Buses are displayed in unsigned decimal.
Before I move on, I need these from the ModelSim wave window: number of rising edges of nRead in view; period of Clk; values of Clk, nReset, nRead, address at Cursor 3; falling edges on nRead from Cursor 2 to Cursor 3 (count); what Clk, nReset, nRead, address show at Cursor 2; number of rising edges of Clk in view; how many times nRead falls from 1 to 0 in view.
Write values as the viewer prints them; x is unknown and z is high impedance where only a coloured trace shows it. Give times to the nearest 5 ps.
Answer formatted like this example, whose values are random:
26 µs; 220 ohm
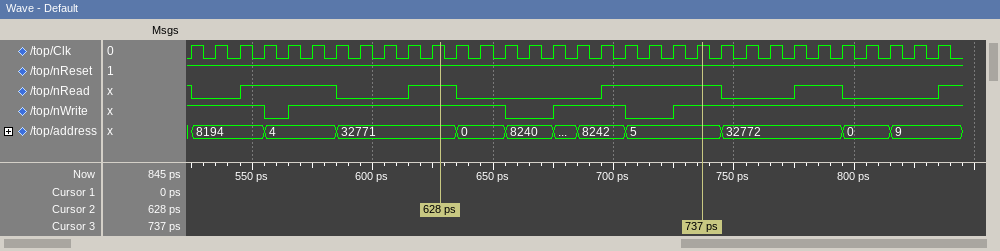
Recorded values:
5; 10 ps; Clk=1, nReset=1, nRead=1, address=5; 1; Clk=1, nReset=1, nRead=1, address=32771; 32; 5
